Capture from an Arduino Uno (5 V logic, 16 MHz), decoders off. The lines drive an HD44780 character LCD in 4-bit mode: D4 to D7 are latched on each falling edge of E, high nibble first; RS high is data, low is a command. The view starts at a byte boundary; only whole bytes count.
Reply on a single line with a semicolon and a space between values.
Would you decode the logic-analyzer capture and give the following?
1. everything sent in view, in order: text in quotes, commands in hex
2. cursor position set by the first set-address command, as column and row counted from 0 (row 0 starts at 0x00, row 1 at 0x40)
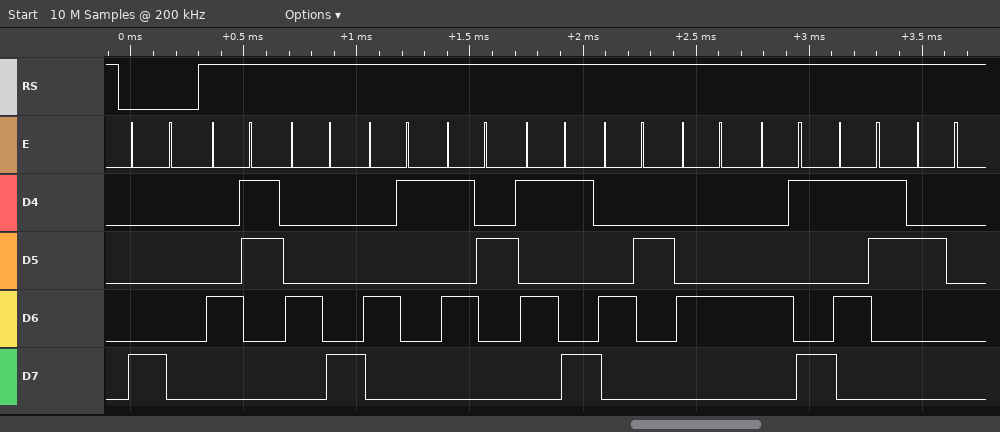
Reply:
0x80 "CHARYBDIS "; column 0, row 0
